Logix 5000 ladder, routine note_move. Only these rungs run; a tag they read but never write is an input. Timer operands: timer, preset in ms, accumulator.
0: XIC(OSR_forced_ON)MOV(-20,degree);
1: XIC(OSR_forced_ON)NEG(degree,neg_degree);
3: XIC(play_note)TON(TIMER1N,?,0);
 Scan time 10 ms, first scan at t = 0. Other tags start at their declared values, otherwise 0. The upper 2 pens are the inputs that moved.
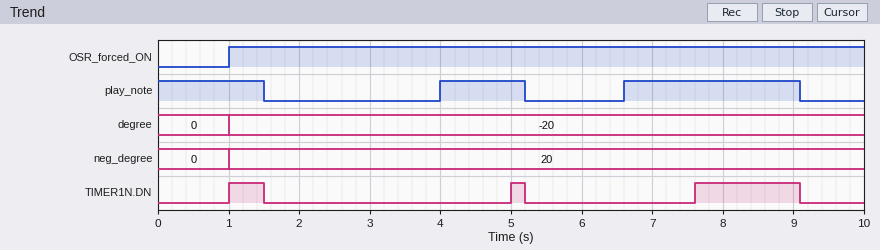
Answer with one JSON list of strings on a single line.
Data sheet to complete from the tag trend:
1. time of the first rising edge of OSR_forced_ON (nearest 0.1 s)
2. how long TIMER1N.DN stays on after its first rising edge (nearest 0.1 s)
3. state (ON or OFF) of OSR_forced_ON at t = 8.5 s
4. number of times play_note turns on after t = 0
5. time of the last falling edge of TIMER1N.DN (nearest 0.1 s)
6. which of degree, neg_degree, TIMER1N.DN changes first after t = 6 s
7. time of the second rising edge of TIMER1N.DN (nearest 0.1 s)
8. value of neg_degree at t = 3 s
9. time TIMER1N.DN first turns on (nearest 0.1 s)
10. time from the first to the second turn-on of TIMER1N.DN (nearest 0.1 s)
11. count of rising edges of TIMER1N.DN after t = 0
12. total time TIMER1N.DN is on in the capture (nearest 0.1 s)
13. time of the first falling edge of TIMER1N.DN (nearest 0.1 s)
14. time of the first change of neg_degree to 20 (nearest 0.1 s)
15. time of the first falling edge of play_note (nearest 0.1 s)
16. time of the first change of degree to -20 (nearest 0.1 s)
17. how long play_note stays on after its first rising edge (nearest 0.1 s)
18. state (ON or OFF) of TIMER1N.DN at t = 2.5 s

["1.0 s", "0.5 s", "ON", "2", "9.1 s", "TIMER1N.DN", "5.0 s", "20", "1.0 s", "4.0 s", "3", "2.2 s", "1.5 s", "1.0 s", "1.5 s", "1.0 s", "1.2 s", "OFF"]
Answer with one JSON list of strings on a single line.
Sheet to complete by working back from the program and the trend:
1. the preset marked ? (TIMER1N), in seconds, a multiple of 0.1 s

["1.0 s"]
